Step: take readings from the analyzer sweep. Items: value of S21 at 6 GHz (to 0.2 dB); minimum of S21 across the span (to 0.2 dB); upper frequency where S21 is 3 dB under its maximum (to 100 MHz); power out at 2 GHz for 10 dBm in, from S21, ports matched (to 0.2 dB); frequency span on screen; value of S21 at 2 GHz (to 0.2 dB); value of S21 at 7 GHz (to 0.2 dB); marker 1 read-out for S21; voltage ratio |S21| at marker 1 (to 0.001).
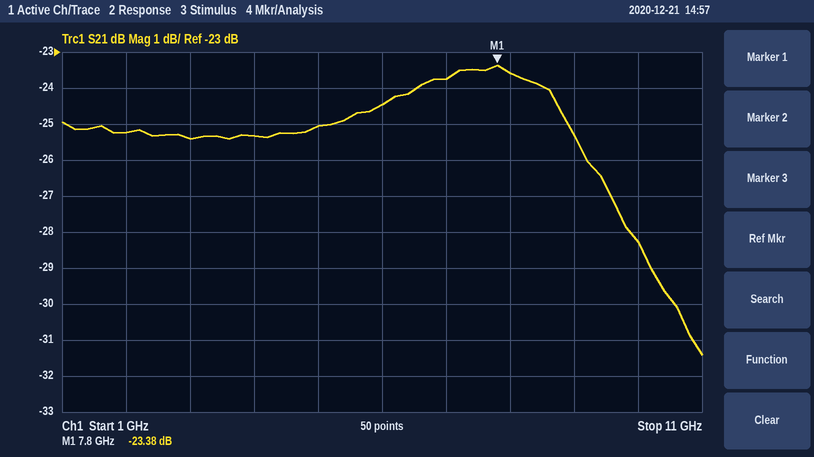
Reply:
-24.4 dB
-31.4 dB
9.4 GHz
-15.2 dBm
10 GHz
-25.2 dB
-23.8 dB
-23.38 dB
0.068
